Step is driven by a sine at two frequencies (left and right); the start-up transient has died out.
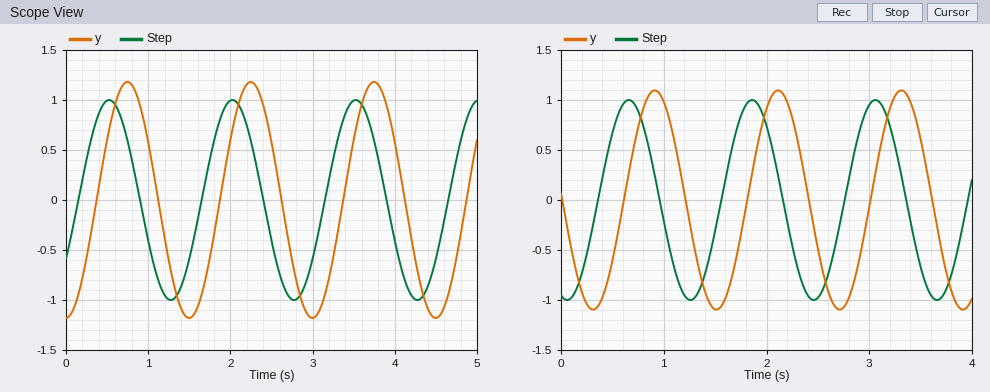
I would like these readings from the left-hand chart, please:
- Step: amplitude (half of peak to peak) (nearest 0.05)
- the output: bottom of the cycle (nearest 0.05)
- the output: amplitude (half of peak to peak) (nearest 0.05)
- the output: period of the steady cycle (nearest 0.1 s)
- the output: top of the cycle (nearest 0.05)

1.00
-1.20
1.20
1.5 s
1.20
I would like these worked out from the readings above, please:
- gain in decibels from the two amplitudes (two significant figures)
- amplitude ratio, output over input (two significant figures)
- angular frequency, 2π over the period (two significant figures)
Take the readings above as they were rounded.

1.6 dB
1.2
4.2 rad/s
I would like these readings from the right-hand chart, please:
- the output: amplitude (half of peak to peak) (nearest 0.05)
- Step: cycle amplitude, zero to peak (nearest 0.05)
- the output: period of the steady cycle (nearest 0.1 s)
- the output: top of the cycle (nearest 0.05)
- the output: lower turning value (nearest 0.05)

1.10
1.00
1.2 s
1.10
-1.10
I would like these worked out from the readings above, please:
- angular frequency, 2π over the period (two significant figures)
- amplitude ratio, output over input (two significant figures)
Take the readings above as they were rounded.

5.2 rad/s
1.1
